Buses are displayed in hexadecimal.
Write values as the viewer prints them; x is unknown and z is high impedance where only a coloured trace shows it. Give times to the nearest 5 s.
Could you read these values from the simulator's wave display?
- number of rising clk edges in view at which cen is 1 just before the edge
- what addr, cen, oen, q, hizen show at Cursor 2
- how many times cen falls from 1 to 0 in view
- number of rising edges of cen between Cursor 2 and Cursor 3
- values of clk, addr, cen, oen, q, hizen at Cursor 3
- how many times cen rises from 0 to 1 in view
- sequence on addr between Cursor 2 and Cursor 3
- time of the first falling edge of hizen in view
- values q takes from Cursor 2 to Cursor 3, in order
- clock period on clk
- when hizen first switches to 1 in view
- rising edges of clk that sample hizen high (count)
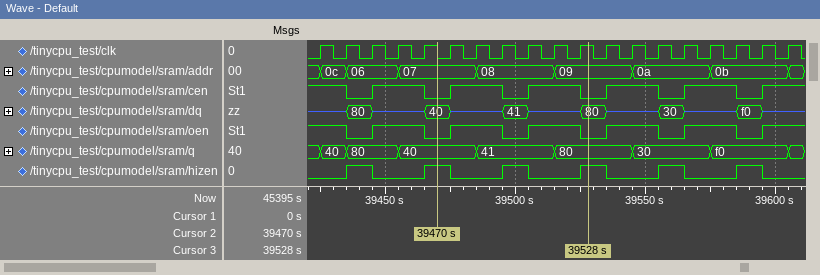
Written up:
13
addr=07, cen=0, oen=0, q=40, hizen=1
6
2
clk=1, addr=09, cen=0, oen=0, q=80, hizen=1
6
07, 08, 09
39445 s
40, 41, 80
10 s
39435 s
6
